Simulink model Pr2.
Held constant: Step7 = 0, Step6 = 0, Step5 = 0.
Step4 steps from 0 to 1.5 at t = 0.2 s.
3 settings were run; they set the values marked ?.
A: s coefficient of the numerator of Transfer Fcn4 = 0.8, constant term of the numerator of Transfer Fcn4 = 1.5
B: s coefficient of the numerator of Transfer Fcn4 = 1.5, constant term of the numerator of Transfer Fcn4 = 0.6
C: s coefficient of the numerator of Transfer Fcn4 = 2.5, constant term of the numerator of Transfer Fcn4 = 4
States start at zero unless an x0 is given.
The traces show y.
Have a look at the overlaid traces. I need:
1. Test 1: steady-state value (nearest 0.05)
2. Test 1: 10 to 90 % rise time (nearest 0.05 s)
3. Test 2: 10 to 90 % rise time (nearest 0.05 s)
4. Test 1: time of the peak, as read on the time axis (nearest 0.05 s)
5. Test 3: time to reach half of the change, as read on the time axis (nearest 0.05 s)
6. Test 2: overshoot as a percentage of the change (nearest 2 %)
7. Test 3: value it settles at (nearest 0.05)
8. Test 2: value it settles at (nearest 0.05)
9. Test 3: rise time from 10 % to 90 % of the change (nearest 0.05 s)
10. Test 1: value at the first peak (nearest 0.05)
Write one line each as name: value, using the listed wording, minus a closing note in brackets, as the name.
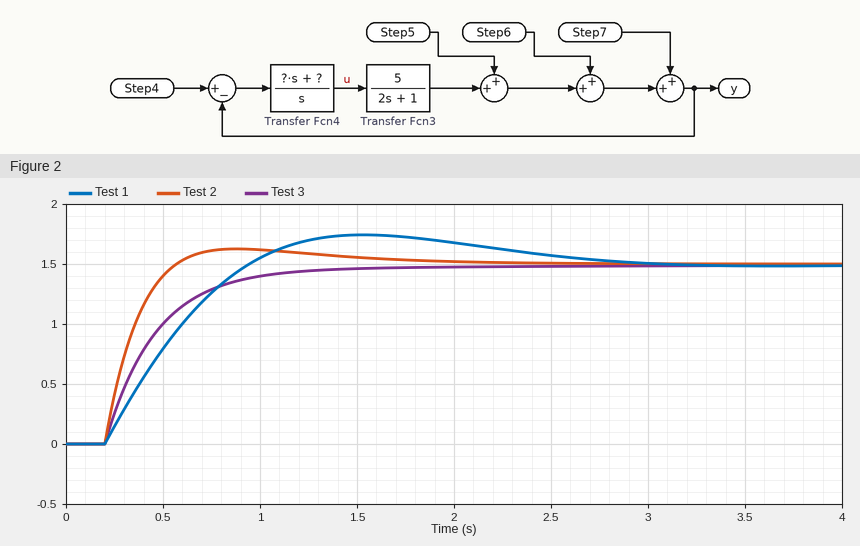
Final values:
Test 1: steady-state value: 1.50
Test 1: 10 to 90 % rise time: 0.55 s
Test 2: 10 to 90 % rise time: 0.25 s
Test 1: time of the peak, as read on the time axis: 1.55 s
Test 3: time to reach half of the change, as read on the time axis: 0.40 s
Test 2: overshoot as a percentage of the change: 8 %
Test 3: value it settles at: 1.50
Test 2: value it settles at: 1.50
Test 3: rise time from 10 % to 90 % of the change: 0.65 s
Test 1: value at the first peak: 1.75
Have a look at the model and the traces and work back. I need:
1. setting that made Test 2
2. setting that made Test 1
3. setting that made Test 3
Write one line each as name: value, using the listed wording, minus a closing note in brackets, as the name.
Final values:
setting that made Test 2: C
setting that made Test 1: A
setting that made Test 3: B
